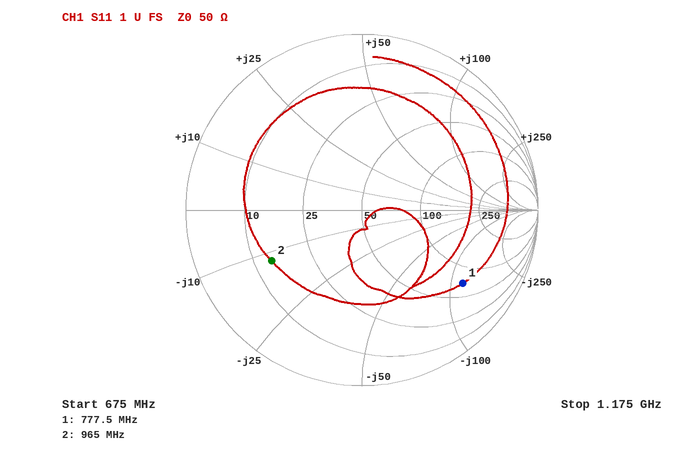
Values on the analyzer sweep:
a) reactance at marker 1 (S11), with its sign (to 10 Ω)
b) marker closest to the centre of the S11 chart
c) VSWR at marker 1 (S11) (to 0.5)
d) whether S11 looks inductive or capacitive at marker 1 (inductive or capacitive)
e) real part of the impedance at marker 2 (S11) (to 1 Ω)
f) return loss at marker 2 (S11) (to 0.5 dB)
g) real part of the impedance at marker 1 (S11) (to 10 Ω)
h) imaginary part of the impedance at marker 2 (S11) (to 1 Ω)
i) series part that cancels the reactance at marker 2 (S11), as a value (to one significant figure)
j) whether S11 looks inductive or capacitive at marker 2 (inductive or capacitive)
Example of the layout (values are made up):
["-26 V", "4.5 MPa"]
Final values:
["-120 Ω", "marker 2", "6.0", "capacitive", "14 Ω", "4.5 dB", "70 Ω", "-12 Ω", "2 nH", "capacitive"]
